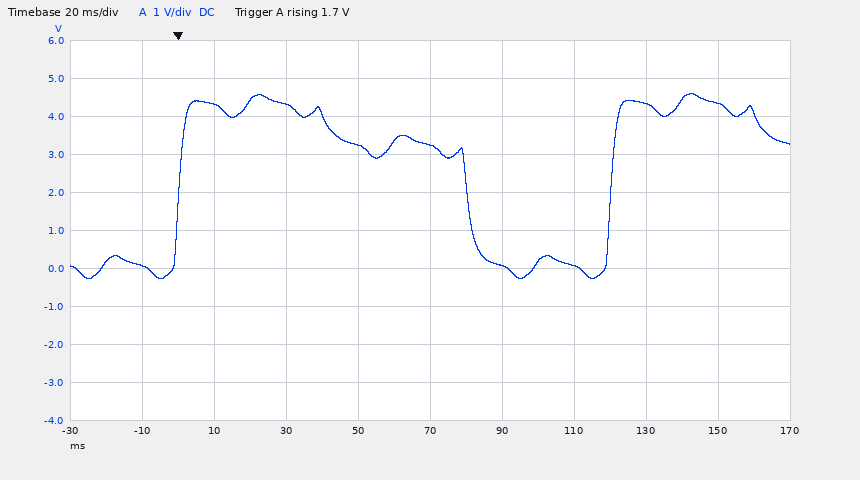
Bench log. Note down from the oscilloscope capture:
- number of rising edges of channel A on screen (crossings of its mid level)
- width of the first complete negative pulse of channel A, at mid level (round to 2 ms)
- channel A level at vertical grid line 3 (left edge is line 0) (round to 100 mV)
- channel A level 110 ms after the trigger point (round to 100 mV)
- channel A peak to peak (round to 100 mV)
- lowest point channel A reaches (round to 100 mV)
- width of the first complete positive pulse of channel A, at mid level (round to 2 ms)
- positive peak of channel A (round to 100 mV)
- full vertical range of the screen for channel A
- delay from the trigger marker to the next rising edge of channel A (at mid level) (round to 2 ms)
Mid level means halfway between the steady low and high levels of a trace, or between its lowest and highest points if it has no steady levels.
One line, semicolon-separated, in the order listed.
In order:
2; 40 ms; 4.3 V; 100 mV; 4.9 V; -300 mV; 80 ms; 4.6 V; 10 V; 120 ms
